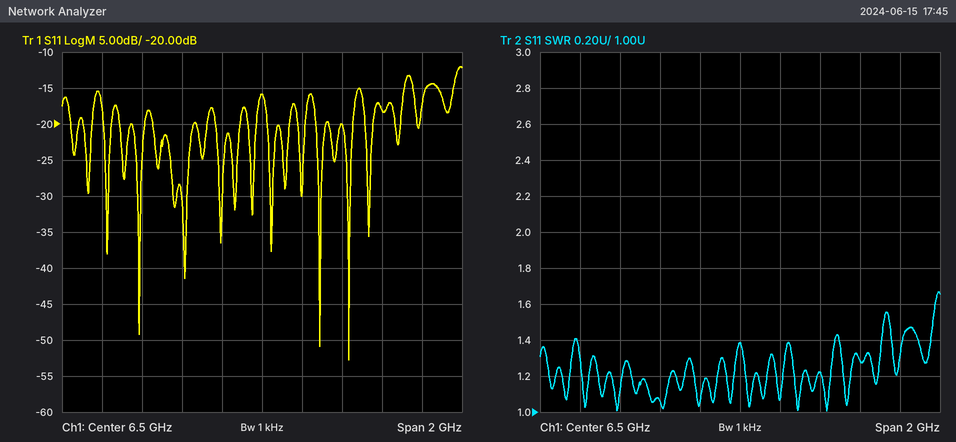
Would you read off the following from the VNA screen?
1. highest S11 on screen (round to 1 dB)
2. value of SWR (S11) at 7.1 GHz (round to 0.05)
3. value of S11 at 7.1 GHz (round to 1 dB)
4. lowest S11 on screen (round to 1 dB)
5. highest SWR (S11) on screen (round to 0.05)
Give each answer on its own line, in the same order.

-12 dB
1.30
-18 dB
-53 dB
1.65
